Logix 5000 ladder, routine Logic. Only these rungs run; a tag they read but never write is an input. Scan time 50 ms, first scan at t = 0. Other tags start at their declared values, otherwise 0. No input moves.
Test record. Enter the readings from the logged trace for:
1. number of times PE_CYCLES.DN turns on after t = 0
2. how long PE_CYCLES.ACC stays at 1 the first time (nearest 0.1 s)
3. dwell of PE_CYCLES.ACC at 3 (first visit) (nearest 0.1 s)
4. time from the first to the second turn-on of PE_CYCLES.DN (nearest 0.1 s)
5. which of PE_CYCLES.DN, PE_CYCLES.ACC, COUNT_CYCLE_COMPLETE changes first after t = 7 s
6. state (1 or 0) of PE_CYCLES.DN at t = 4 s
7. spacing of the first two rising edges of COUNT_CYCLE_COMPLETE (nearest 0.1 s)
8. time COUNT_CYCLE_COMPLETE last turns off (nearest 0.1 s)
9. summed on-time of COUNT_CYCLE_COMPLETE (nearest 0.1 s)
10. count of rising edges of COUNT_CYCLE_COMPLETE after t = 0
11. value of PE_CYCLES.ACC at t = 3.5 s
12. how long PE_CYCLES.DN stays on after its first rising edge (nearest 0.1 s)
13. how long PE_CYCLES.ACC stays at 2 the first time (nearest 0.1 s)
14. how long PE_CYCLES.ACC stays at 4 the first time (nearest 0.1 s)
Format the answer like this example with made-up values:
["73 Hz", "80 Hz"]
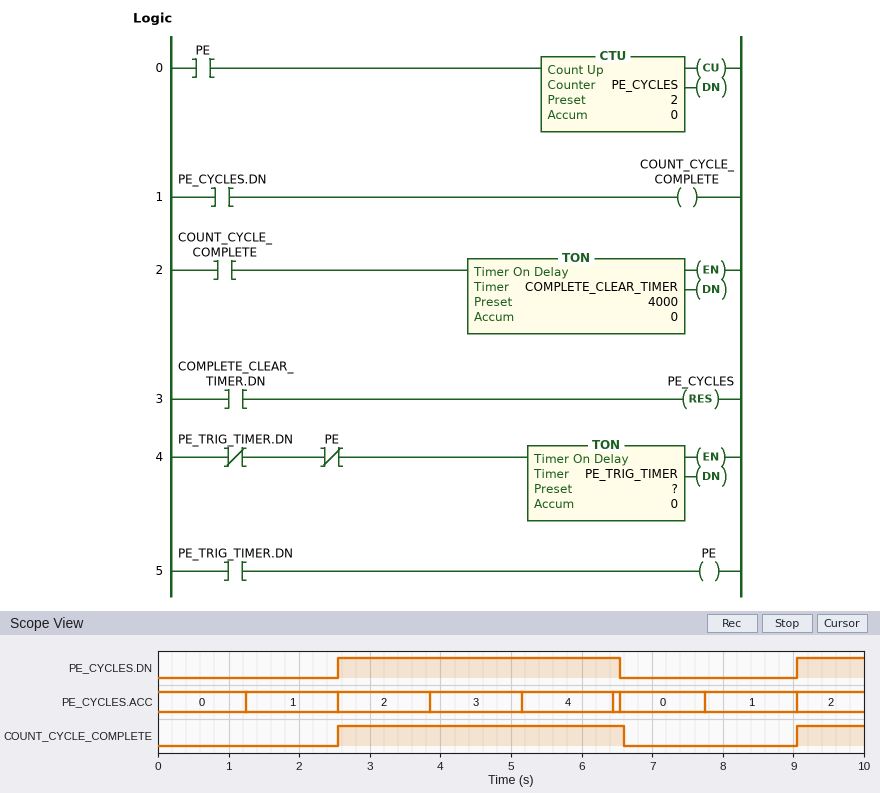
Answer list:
["2", "1.3 s", "1.3 s", "6.5 s", "PE_CYCLES.ACC", "1", "6.5 s", "6.6 s", "5.0 s", "2", "2", "4.0 s", "1.3 s", "1.3 s"]
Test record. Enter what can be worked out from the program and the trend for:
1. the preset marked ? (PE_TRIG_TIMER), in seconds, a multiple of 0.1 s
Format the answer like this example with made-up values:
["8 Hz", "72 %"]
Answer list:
["1.2 s"]
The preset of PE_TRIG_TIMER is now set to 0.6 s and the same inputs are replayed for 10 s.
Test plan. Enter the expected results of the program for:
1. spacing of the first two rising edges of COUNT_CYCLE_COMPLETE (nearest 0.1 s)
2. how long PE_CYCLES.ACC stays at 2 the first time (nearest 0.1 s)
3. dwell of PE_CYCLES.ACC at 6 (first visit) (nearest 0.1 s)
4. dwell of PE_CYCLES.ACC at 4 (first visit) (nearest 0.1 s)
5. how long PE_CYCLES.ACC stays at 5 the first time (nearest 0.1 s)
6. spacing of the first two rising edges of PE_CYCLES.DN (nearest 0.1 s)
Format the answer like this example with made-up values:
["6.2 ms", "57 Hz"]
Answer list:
["4.9 s", "0.7 s", "0.7 s", "0.7 s", "0.7 s", "4.9 s"]
